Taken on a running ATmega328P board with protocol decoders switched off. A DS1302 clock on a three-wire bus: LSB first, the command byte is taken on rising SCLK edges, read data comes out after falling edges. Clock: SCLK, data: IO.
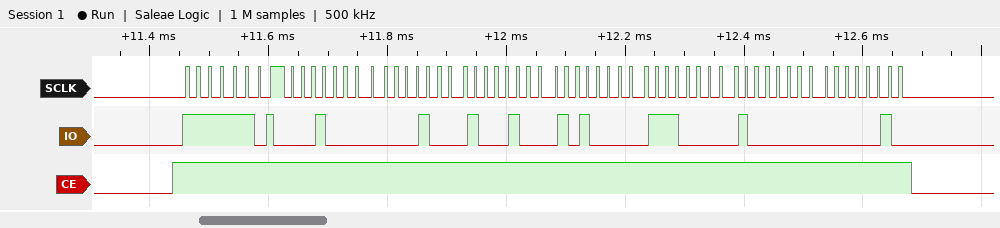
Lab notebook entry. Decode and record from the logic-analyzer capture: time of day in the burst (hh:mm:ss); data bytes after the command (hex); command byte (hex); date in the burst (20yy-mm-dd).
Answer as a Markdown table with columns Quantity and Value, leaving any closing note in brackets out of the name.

| Quantity | Value |
|---|---|
| time of day in the burst | 11:10:08 |
| data bytes after the command | 08 10 11 05 07 01 20 |
| command byte | 0xBF |
| date in the burst | 2020-07-05 |
